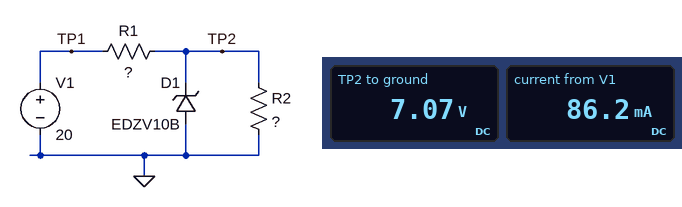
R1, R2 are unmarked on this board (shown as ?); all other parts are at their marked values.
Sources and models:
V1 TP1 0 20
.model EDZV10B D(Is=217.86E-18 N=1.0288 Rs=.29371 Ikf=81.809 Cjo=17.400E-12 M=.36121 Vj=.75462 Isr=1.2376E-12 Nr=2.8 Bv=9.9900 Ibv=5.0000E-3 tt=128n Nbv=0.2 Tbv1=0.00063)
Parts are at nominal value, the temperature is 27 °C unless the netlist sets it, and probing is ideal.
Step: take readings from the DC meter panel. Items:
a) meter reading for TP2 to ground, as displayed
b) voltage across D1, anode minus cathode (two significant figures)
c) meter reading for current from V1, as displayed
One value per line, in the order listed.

7.07 V
-7.1 V
86.2 mA
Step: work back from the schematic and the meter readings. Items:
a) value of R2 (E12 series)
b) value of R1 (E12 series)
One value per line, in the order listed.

82 Ω
150 Ω
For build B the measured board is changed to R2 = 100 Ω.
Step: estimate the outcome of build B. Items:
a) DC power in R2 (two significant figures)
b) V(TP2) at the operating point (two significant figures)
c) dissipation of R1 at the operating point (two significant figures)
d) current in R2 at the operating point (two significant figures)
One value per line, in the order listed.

640 mW
8.0 V
960 mW
80 mA
